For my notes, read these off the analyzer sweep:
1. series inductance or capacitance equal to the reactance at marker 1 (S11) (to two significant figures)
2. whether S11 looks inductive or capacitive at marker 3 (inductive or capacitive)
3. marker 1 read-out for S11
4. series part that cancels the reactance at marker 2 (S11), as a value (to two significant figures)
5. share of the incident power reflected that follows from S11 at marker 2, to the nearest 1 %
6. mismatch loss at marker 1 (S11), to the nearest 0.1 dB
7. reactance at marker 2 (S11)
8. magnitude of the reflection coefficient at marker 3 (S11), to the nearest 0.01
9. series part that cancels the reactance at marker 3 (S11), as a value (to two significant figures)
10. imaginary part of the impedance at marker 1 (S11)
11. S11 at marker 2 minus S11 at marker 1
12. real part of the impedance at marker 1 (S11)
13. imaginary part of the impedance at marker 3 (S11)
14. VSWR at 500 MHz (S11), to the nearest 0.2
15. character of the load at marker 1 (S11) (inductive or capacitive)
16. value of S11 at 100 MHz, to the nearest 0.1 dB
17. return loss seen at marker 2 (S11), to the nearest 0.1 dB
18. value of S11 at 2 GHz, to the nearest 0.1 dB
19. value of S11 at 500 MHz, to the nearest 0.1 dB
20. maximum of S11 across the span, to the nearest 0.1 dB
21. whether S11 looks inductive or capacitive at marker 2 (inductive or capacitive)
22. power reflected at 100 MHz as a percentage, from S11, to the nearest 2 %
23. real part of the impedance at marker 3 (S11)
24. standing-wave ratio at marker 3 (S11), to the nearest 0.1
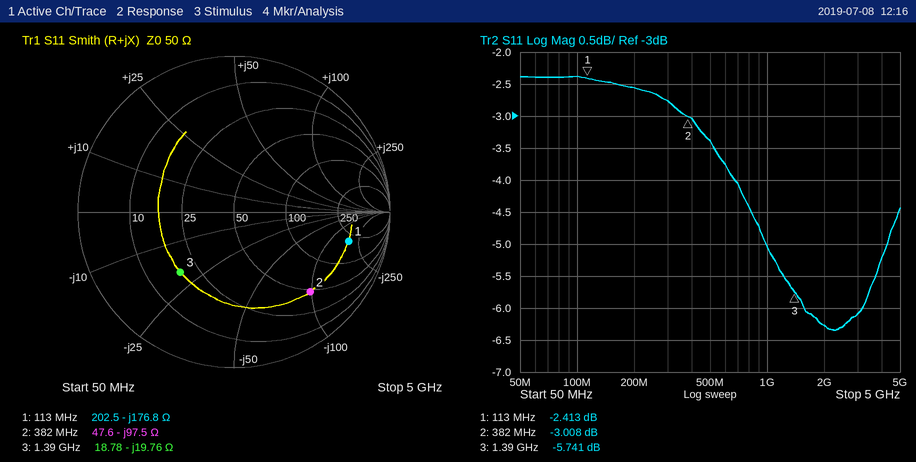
8.0 pF
capacitive
-2.413 dB
41 nH
50 %
3.7 dB
-97.5 Ω
0.52
2.3 nH
-176.8 Ω
-0.595 dB
202.5 Ω
-19.76 Ω
5.2
capacitive
-2.4 dB
3.0 dB
-6.3 dB
-3.4 dB
-2.4 dB
capacitive
58 %
18.78 Ω
3.1
